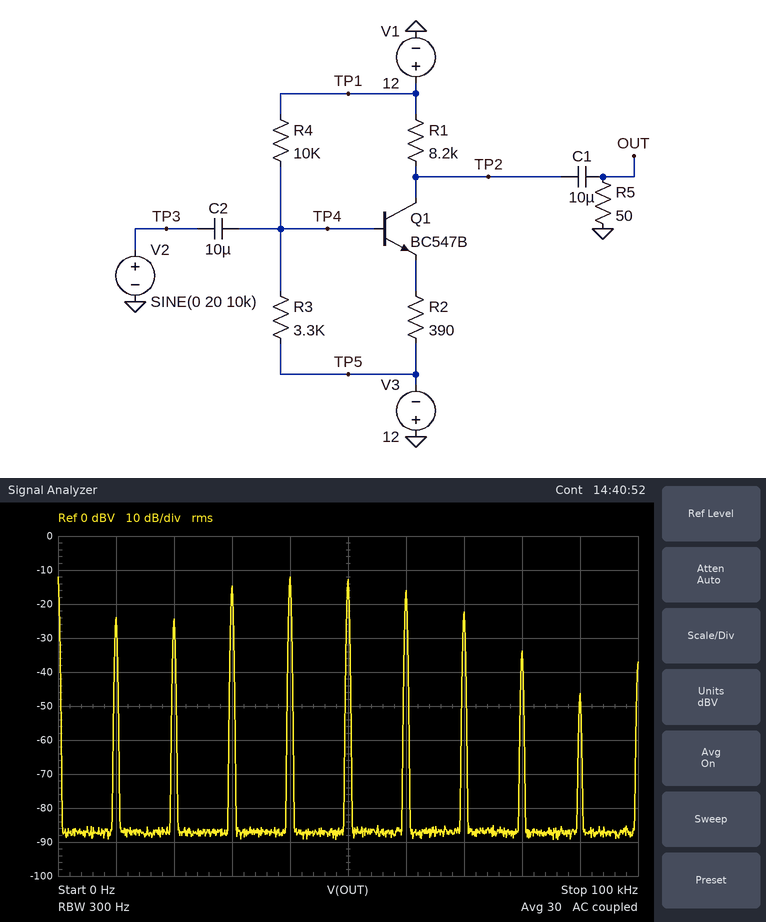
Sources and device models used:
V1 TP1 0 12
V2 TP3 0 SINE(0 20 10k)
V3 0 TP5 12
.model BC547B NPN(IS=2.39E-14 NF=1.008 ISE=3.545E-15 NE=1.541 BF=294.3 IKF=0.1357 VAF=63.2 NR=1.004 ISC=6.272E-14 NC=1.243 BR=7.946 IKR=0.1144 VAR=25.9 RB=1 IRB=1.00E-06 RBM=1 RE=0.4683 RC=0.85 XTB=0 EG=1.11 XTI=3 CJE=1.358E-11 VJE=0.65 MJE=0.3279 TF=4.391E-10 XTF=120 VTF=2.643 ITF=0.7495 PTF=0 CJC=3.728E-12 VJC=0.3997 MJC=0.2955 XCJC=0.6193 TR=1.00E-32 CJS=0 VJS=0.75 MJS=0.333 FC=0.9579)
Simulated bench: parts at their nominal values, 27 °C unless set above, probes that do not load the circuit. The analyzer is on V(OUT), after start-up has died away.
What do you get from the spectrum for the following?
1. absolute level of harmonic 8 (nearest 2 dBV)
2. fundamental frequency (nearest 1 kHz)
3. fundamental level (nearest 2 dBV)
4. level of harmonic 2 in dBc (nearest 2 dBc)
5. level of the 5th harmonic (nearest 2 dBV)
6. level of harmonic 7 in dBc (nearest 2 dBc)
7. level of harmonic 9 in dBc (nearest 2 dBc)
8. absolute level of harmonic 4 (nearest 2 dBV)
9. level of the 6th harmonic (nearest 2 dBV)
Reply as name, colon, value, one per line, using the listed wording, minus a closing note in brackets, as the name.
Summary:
absolute level of harmonic 8: -34 dBV
fundamental frequency: 10 kHz
fundamental level: -24 dBV
level of harmonic 2 in dBc: 0 dBc
level of the 5th harmonic: -12 dBV
level of harmonic 7 in dBc: 2 dBc
level of harmonic 9 in dBc: -22 dBc
absolute level of harmonic 4: -12 dBV
level of the 6th harmonic: -16 dBV
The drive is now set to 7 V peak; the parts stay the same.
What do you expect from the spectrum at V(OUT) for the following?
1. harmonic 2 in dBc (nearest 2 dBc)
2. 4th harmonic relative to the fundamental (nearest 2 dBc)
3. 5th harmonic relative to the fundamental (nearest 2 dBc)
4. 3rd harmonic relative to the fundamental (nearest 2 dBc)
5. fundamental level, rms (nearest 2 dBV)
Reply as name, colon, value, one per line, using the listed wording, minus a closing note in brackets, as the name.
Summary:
harmonic 2 in dBc: -14 dBc
4th harmonic relative to the fundamental: 2 dBc
5th harmonic relative to the fundamental: -2 dBc
3rd harmonic relative to the fundamental: 2 dBc
fundamental level, rms: -20 dBV
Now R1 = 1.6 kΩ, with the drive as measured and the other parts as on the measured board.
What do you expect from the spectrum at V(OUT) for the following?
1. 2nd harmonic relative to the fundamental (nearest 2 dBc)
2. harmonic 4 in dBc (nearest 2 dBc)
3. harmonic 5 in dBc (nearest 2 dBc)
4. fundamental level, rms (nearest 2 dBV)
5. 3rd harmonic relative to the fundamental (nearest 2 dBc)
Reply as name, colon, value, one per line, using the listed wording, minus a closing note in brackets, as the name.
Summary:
2nd harmonic relative to the fundamental: -12 dBc
harmonic 4 in dBc: -2 dBc
harmonic 5 in dBc: -4 dBc
fundamental level, rms: -10 dBV
3rd harmonic relative to the fundamental: -6 dBc
